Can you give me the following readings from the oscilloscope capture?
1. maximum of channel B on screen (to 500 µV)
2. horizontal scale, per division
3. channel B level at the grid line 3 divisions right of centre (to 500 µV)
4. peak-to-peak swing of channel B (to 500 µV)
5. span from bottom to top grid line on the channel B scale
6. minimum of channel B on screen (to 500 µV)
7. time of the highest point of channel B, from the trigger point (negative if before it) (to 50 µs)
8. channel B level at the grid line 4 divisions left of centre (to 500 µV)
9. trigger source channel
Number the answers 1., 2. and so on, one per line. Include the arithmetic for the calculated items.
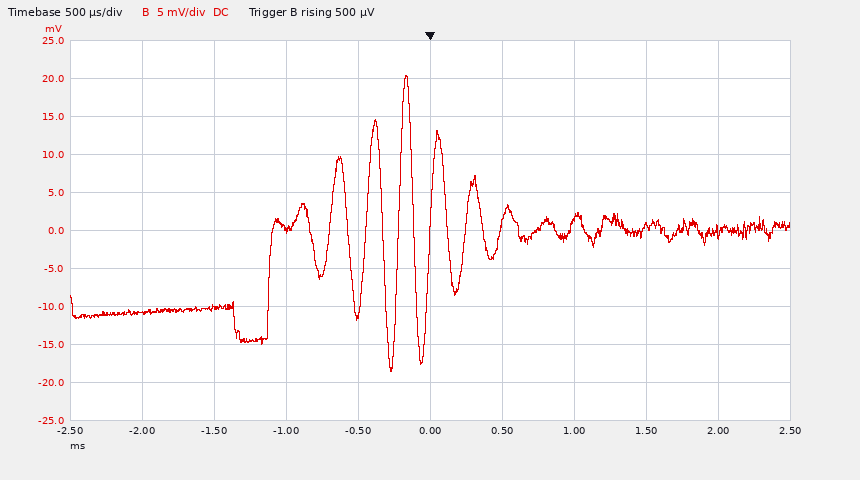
1. 20.5 mV
2. 500 µs
3. 500 µV
4. 20.5 mV − (-18.5 mV) = 39.0 mV
5. 50 mV
6. -18.5 mV
7. -150 µs
8. -11.0 mV
9. channel B
